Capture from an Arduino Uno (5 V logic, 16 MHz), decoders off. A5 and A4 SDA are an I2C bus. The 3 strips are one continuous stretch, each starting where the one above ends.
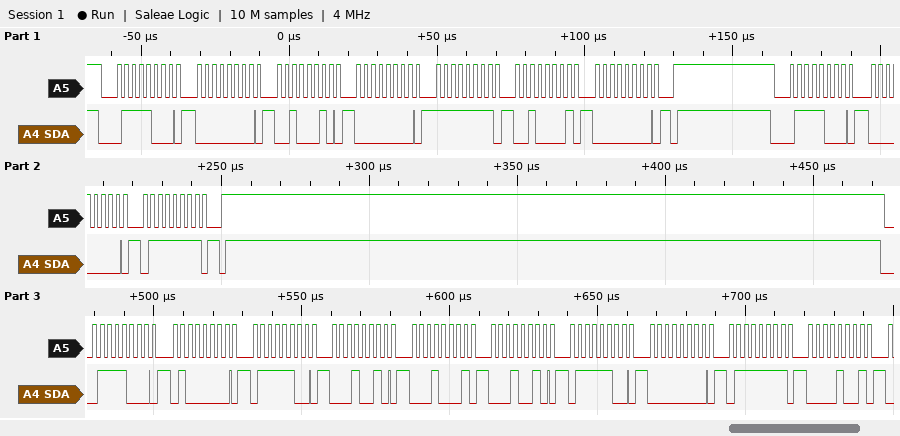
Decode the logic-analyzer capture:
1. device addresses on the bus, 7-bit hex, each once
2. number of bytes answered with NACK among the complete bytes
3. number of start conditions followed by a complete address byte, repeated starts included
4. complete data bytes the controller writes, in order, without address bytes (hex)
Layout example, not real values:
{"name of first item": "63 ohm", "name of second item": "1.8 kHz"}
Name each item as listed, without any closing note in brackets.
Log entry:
{"device addresses on the bus, 7-bit hex, each once": "0x3C", "number of bytes answered with NACK among the complete bytes": "0", "number of start conditions followed by a complete address byte, repeated starts included": "3", "complete data bytes the controller writes, in order, without address bytes": "00 22 00 FF 21 00 00 7F 40 7C 12 11 12 7C 00 7F 09"}
